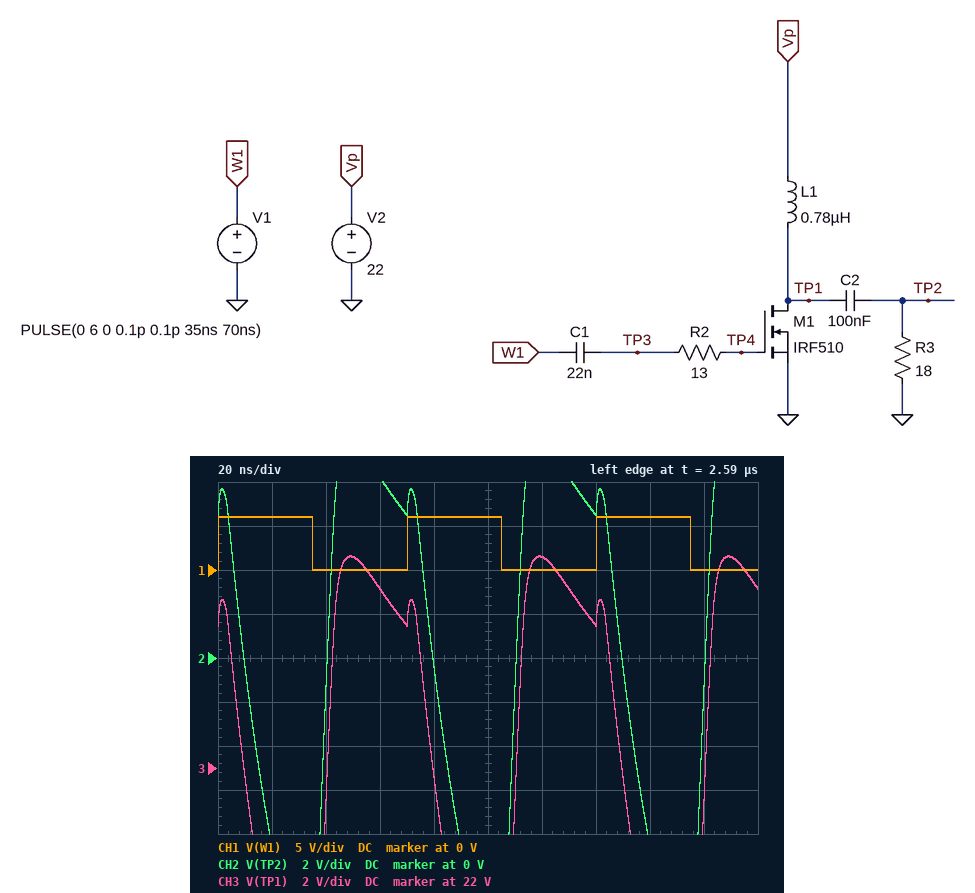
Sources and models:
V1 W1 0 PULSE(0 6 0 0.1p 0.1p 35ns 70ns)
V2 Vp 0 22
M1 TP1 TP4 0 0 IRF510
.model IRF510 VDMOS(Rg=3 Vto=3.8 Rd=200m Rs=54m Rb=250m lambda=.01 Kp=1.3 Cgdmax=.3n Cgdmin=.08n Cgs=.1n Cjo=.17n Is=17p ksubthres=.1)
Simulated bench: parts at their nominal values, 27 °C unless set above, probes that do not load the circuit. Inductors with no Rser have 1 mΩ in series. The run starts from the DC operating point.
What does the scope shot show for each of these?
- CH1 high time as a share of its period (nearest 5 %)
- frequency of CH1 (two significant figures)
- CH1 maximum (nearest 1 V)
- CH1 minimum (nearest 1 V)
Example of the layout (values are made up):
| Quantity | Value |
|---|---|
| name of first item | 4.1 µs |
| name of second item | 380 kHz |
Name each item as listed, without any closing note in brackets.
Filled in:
| Quantity | Value |
|---|---|
| CH1 high time as a share of its period | 50 % |
| frequency of CH1 | 14 MHz |
| CH1 maximum | 6 V |
| CH1 minimum | 0 V |
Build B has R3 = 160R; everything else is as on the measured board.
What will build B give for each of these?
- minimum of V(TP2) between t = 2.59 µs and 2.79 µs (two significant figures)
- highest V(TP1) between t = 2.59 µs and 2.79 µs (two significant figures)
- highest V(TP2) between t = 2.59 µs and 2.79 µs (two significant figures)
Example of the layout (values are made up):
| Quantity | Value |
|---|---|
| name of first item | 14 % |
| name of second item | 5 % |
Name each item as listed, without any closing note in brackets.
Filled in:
| Quantity | Value |
|---|---|
| minimum of V(TP2) between t = 2.59 µs and 2.79 µs | -11 V |
| highest V(TP1) between t = 2.59 µs and 2.79 µs | 47 V |
| highest V(TP2) between t = 2.59 µs and 2.79 µs | 35 V |
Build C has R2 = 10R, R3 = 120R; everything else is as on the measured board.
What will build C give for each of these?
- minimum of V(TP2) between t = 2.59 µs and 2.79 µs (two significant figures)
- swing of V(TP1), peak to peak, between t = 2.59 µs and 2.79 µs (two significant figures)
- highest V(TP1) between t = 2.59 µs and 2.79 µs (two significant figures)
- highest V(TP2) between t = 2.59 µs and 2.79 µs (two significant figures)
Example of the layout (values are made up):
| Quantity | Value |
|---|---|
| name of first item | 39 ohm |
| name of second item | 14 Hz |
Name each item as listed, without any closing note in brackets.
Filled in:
| Quantity | Value |
|---|---|
| minimum of V(TP2) between t = 2.59 µs and 2.79 µs | -21 V |
| swing of V(TP1), peak to peak, between t = 2.59 µs and 2.79 µs | 47 V |
| highest V(TP1) between t = 2.59 µs and 2.79 µs | 48 V |
| highest V(TP2) between t = 2.59 µs and 2.79 µs | 26 V |
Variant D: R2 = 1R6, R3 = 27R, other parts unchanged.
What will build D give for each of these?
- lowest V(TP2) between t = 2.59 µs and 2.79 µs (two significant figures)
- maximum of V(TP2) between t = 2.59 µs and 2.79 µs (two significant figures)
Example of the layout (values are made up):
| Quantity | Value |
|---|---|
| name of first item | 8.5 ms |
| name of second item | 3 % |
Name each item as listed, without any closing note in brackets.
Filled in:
| Quantity | Value |
|---|---|
| lowest V(TP2) between t = 2.59 µs and 2.79 µs | -21 V |
| maximum of V(TP2) between t = 2.59 µs and 2.79 µs | 23 V |
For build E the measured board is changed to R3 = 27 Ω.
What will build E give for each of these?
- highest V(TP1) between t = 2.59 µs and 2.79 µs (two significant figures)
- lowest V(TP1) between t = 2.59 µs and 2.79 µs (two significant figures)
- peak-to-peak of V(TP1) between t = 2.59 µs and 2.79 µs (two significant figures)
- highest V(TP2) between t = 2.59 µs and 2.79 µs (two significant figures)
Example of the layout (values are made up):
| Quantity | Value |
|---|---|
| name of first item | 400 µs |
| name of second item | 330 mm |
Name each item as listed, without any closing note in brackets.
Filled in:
| Quantity | Value |
|---|---|
| highest V(TP1) between t = 2.59 µs and 2.79 µs | 34 V |
| lowest V(TP1) between t = 2.59 µs and 2.79 µs | 5.2 V |
| peak-to-peak of V(TP1) between t = 2.59 µs and 2.79 µs | 29 V |
| highest V(TP2) between t = 2.59 µs and 2.79 µs | 12 V |
